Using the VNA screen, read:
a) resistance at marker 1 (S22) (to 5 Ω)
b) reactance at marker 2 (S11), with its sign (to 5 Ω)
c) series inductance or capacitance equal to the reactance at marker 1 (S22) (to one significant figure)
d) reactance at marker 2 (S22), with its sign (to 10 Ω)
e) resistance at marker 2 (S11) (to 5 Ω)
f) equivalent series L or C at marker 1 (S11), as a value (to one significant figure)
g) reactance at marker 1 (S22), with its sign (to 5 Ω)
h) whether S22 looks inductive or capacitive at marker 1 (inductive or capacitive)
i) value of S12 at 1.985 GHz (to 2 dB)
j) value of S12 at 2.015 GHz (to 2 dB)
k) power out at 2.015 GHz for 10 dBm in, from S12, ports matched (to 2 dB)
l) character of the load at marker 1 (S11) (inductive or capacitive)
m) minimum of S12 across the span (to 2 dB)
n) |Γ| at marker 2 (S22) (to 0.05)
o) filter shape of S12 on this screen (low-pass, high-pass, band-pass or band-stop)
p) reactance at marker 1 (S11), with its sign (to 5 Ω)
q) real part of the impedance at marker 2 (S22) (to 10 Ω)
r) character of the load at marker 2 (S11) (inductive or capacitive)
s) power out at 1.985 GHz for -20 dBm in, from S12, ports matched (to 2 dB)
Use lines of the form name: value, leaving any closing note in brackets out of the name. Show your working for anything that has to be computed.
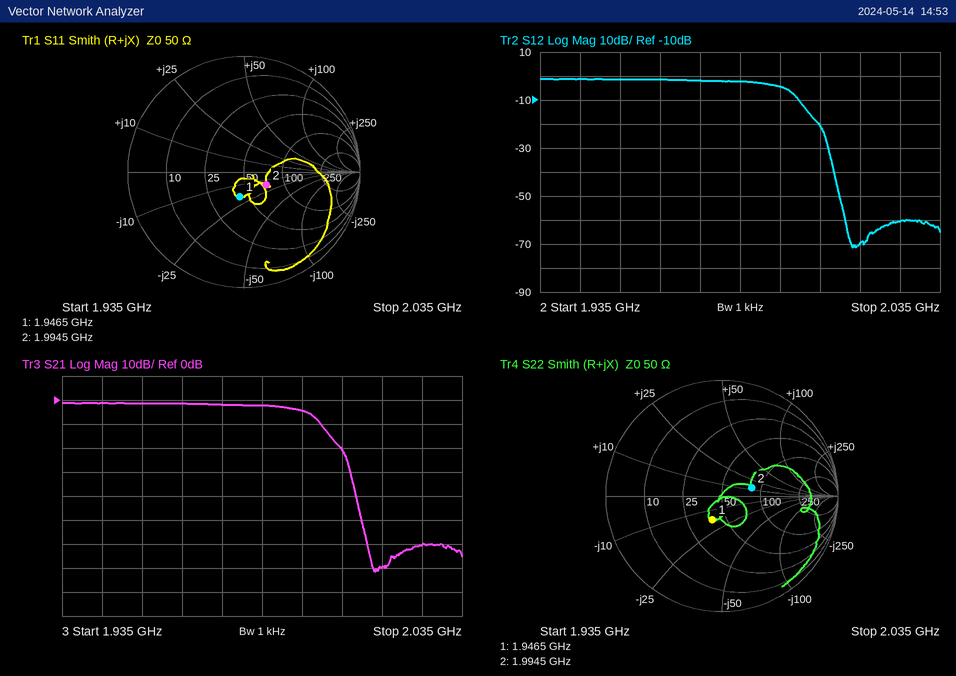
resistance at marker 1 (S22): 40 Ω
reactance at marker 2 (S11), with its sign: -15 Ω
series inductance or capacitance equal to the reactance at marker 1 (S22): C = 1/(2π × 1.9465 GHz × 15 Ω) ≈ 5 pF
reactance at marker 2 (S22), with its sign: +10 Ω
resistance at marker 2 (S11): 70 Ω
equivalent series L or C at marker 1 (S11), as a value: C = 1/(2π × 1.9465 GHz × 20 Ω) ≈ 4 pF
reactance at marker 1 (S22), with its sign: -15 Ω
whether S22 looks inductive or capacitive at marker 1: capacitive
value of S12 at 1.985 GHz: -2 dB
value of S12 at 2.015 GHz: -70 dB
power out at 2.015 GHz for 10 dBm in, from S12, ports matched: 10 dBm + (-70 dB) = -60 dBm
character of the load at marker 1 (S11): capacitive
minimum of S12 across the span: -72 dB
|Γ| at marker 2 (S22): 0.25
filter shape of S12 on this screen: low-pass
reactance at marker 1 (S11), with its sign: -20 Ω
real part of the impedance at marker 2 (S22): 80 Ω
character of the load at marker 2 (S11): capacitive
power out at 1.985 GHz for -20 dBm in, from S12, ports matched: -20 dBm + (-2 dB) = -22 dBm
